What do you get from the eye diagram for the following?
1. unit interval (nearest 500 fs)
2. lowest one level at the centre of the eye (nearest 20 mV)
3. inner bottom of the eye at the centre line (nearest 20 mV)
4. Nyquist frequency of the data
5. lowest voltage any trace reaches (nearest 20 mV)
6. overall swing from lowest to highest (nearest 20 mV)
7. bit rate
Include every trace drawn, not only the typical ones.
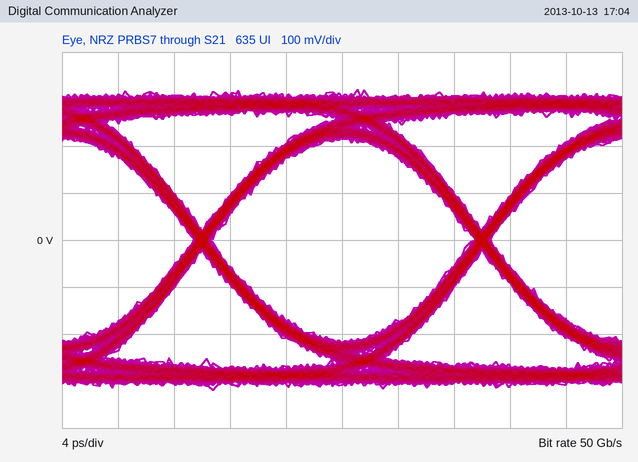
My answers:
20.0 ps
220 mV
-220 mV
25 GHz
-320 mV
640 mV
50 Gb/s
